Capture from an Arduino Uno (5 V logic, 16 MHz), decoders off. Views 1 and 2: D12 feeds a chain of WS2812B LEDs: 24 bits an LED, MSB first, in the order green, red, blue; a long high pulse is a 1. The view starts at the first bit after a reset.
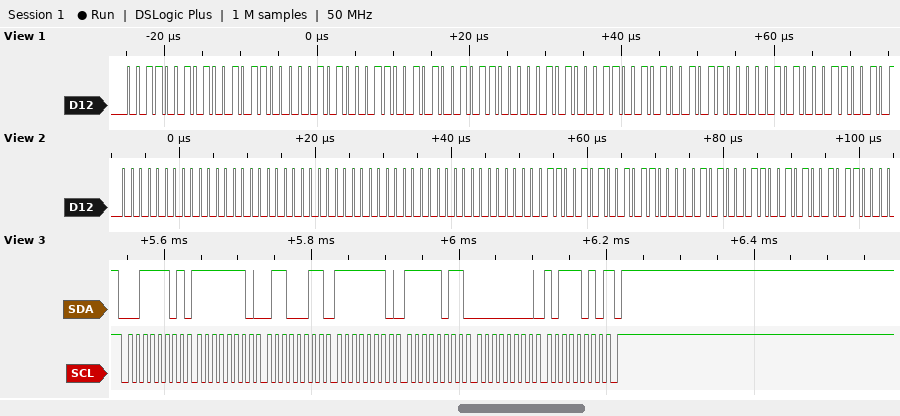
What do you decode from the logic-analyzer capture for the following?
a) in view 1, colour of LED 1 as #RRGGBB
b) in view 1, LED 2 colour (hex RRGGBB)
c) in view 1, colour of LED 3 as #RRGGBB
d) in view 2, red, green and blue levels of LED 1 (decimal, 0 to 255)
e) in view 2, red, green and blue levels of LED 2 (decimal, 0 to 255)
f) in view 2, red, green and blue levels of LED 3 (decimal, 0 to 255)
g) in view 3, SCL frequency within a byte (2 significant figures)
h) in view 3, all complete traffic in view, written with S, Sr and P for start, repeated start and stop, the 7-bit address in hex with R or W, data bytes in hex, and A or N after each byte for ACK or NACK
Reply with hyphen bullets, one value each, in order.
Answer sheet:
- #96320A
- #96320A
- #96320A
- 0, 0, 0
- 0, 0, 0
- 150, 50, 10
- 100 kHz
- S 1ER A FE A 63 A FE A FB A 00 A BA N P
